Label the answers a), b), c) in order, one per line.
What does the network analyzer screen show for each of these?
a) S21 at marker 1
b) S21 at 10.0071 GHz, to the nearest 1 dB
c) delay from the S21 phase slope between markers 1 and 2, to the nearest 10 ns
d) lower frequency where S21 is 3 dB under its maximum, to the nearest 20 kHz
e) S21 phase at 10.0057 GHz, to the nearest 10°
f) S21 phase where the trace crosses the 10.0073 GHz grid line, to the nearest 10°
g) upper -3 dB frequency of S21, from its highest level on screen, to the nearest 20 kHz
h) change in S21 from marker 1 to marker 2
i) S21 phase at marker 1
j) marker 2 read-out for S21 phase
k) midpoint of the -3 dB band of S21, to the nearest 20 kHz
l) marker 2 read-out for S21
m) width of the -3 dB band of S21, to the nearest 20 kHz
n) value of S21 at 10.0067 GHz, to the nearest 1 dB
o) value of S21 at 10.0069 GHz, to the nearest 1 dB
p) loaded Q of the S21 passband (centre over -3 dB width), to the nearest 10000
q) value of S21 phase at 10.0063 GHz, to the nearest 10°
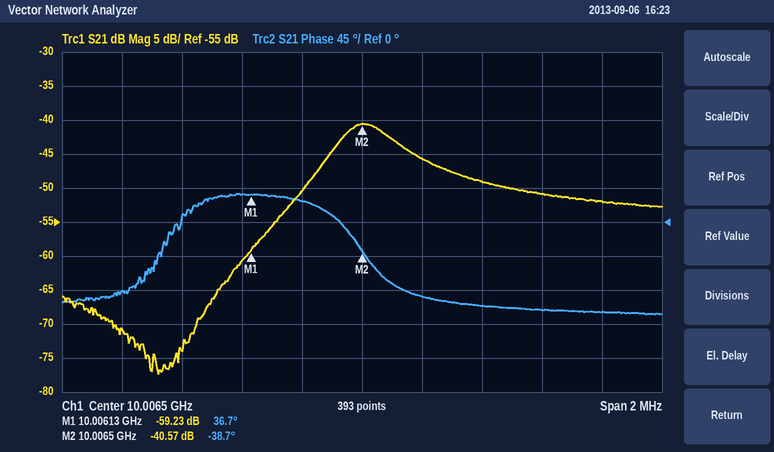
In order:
a) -59.23 dB
b) -51 dB
c) 570 ns
d) 10.00642 GHz
e) -90°
f) -120°
g) 10.00662 GHz
h) 18.66 dB
i) 36.7°
j) -38.7°
k) 10.00652 GHz
l) -40.57 dB
m) 200 kHz
n) -46 dB
o) -49 dB
p) 50000
q) 30°
